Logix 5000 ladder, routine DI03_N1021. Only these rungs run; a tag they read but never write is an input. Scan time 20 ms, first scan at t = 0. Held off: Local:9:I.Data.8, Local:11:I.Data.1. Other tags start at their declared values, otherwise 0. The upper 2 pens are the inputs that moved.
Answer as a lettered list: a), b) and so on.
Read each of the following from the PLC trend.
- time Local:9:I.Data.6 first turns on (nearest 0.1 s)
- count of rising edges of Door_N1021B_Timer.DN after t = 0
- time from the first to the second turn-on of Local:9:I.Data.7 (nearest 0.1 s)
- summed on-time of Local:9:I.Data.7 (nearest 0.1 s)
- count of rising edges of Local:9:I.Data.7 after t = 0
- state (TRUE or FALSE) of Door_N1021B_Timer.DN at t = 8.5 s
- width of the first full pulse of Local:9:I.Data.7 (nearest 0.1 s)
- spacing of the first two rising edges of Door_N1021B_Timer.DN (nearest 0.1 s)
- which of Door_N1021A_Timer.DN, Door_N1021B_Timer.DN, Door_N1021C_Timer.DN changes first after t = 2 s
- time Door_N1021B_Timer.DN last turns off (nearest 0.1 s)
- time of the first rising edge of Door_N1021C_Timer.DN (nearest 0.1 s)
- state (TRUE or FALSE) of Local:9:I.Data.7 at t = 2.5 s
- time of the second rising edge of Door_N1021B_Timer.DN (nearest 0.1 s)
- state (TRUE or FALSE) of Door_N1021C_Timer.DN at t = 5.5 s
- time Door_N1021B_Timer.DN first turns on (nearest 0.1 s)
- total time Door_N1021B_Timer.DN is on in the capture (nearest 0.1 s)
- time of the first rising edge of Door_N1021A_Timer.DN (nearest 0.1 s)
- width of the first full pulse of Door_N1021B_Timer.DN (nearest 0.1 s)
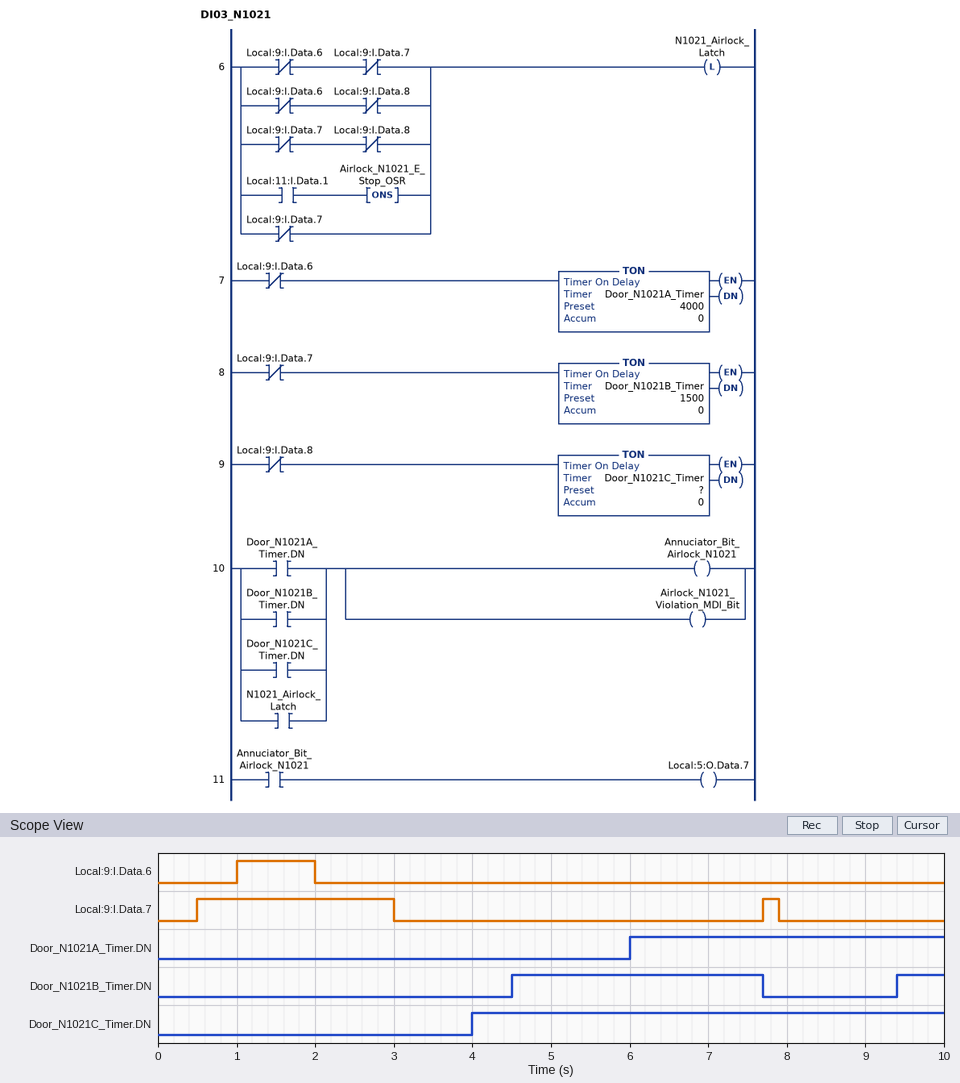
a) 1.0 s
b) 2
c) 7.2 s
d) 2.7 s
e) 2
f) FALSE
g) 2.5 s
h) 4.9 s
i) Door_N1021C_Timer.DN
j) 7.7 s
k) 4.0 s
l) TRUE
m) 9.4 s
n) TRUE
o) 4.5 s
p) 3.8 s
q) 6.0 s
r) 3.2 s
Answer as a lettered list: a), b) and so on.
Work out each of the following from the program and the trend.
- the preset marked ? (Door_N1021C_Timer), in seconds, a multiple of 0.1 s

a) 4.0 s
